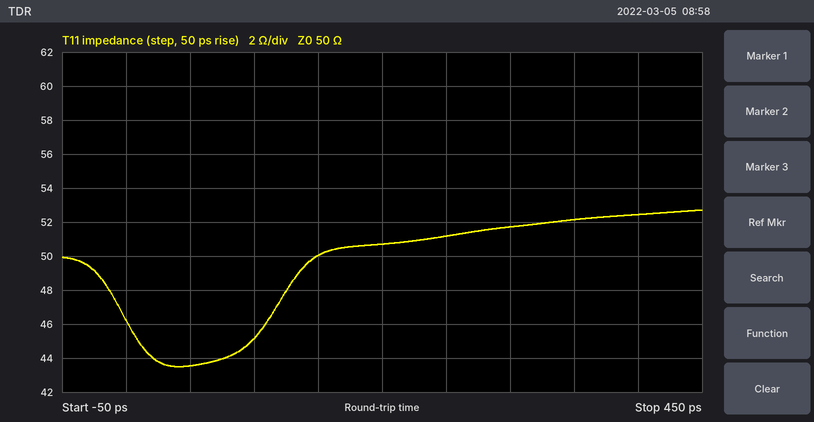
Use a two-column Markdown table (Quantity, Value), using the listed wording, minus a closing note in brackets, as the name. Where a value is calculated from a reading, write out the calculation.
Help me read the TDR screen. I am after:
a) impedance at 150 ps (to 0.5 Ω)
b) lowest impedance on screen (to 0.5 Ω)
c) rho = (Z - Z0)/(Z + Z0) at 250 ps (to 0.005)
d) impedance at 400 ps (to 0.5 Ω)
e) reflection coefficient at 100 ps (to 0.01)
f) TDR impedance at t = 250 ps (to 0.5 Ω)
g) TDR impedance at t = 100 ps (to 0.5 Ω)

| Quantity | Value |
|---|---|
| impedance at 150 ps | 50.0 Ω |
| lowest impedance on screen | 43.5 Ω |
| rho = (Z - Z0)/(Z + Z0) at 250 ps | (51 − 50)/(51 + 50) ≈ +0.010 |
| impedance at 400 ps | 52.5 Ω |
| reflection coefficient at 100 ps | (45 − 50)/(45 + 50) ≈ -0.05 |
| TDR impedance at t = 250 ps | 51.0 Ω |
| TDR impedance at t = 100 ps | 45.0 Ω |
